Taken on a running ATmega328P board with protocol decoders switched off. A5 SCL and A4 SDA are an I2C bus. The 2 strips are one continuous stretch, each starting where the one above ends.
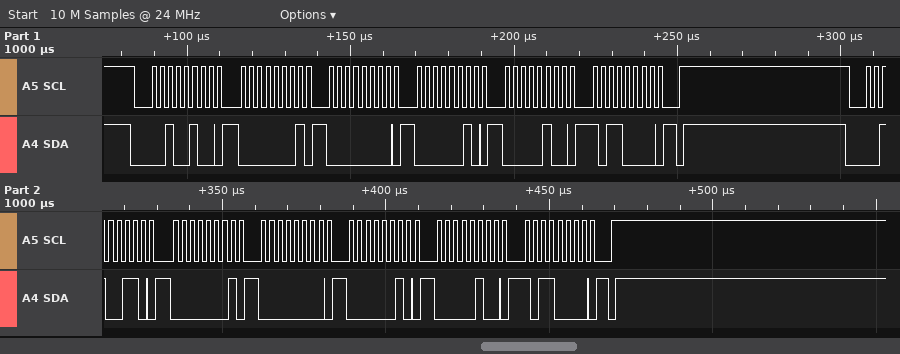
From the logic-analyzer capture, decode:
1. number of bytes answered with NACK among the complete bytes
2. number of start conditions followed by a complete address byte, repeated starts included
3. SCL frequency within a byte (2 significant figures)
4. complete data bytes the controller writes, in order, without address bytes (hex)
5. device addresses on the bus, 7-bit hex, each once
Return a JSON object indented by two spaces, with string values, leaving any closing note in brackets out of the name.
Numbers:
{
  "number of bytes answered with NACK among the complete bytes": "0",
  "number of start conditions followed by a complete address byte, repeated starts included": "2",
  "SCL frequency within a byte": "400 kHz",
  "complete data bytes the controller writes, in order, without address bytes": "01 00 02 04 B0 01 00 02 04 B0",
  "device addresses on the bus, 7-bit hex, each once": "0x12 0x13"
}
